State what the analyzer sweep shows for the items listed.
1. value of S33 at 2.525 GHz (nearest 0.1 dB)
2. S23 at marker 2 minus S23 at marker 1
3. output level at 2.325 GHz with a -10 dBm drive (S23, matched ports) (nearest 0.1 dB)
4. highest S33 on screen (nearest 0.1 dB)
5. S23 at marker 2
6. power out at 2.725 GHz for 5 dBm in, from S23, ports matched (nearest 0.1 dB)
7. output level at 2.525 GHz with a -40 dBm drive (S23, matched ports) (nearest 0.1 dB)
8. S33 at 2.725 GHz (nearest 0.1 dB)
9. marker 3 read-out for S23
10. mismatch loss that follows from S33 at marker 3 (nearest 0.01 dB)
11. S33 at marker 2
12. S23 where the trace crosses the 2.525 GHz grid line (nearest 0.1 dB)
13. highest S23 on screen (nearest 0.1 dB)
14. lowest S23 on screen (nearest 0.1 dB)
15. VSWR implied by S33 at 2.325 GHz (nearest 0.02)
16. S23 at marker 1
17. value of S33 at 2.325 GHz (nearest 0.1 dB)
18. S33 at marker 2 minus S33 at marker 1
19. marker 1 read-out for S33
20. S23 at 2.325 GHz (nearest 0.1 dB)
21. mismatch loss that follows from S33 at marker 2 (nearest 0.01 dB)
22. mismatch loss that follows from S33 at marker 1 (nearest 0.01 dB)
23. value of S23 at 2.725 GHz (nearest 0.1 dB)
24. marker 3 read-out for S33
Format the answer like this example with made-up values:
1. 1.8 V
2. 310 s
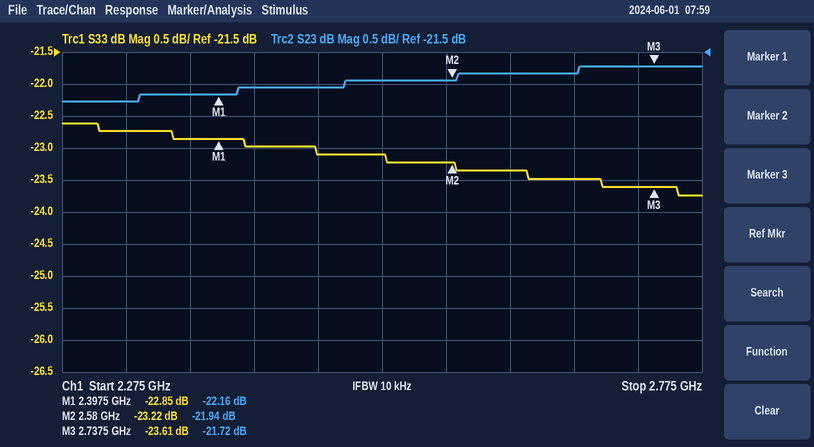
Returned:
1. -23.1 dB
2. 0.22 dB
3. -32.3 dBm
4. -22.6 dB
5. -21.94 dB
6. -16.7 dBm
7. -61.9 dBm
8. -23.6 dB
9. -21.72 dB
10. 0.02 dB
11. -23.22 dB
12. -21.9 dB
13. -21.7 dB
14. -22.3 dB
15. 1.16
16. -22.16 dB
17. -22.7 dB
18. -0.37 dB
19. -22.85 dB
20. -22.3 dB
21. 0.02 dB
22. 0.02 dB
23. -21.7 dB
24. -23.61 dB
